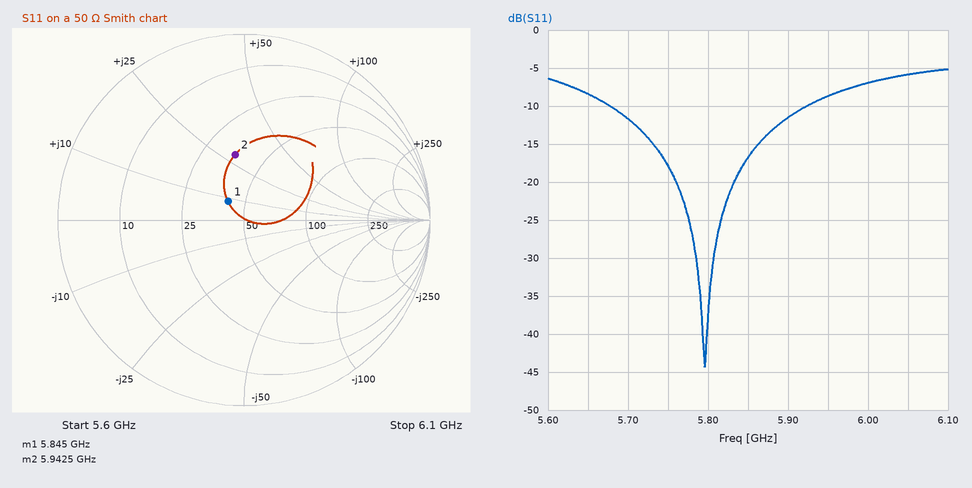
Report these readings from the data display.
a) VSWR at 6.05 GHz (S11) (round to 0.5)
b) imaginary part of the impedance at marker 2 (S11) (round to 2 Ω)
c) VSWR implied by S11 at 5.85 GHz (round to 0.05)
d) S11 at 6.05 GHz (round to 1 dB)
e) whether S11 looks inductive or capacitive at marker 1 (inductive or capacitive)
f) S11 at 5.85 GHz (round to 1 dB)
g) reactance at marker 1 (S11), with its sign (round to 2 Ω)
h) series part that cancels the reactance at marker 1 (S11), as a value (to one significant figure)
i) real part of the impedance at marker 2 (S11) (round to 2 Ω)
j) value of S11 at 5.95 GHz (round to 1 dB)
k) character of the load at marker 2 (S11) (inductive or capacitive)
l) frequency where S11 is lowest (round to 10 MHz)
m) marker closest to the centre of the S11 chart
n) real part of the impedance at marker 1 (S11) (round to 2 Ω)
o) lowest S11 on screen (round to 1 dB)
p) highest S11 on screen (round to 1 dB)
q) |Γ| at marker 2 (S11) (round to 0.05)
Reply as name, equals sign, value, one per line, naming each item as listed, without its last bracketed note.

VSWR at 6.05 GHz (S11) = 3.0
imaginary part of the impedance at marker 2 (S11) = +28 Ω
VSWR implied by S11 at 5.85 GHz = 1.35
S11 at 6.05 GHz = -6 dB
whether S11 looks inductive or capacitive at marker 1 = inductive
S11 at 5.85 GHz = -17 dB
reactance at marker 1 (S11), with its sign = +8 Ω
series part that cancels the reactance at marker 1 (S11), as a value = 3 pF
real part of the impedance at marker 2 (S11) = 36 Ω
value of S11 at 5.95 GHz = -9 dB
character of the load at marker 2 (S11) = inductive
frequency where S11 is lowest = 5.80 GHz
marker closest to the centre of the S11 chart = marker 1
real part of the impedance at marker 1 (S11) = 42 Ω
lowest S11 on screen = -44 dB
highest S11 on screen = -5 dB
|Γ| at marker 2 (S11) = 0.35
